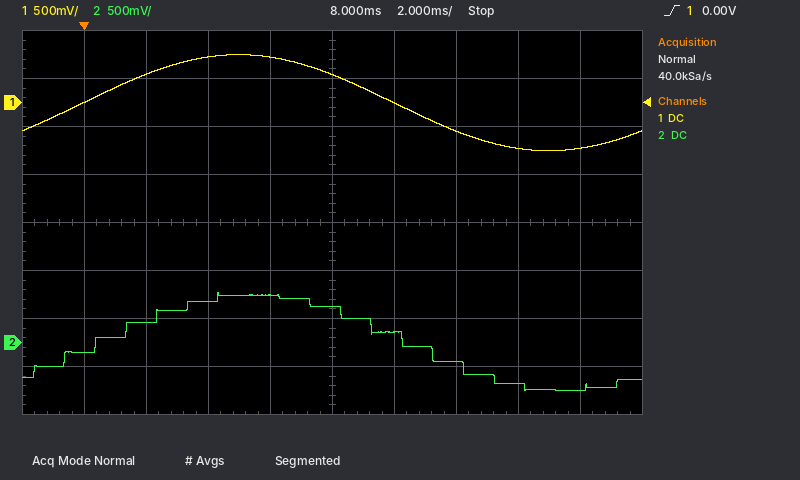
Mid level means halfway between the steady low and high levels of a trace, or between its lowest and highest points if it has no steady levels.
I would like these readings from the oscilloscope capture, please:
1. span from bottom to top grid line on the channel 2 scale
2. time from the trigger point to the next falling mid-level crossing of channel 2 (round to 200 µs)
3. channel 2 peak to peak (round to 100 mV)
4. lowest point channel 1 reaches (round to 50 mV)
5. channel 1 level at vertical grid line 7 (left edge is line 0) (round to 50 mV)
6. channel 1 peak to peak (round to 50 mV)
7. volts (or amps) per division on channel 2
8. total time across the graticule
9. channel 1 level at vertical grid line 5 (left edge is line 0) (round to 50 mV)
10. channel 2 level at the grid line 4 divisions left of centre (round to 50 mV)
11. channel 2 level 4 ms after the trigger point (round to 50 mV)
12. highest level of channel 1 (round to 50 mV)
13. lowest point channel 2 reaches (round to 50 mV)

4 V
10.2 ms
1.00 V
-500 mV
-300 mV
1.00 V
500 mV
20 ms
300 mV
-100 mV
450 mV
500 mV
-500 mV
